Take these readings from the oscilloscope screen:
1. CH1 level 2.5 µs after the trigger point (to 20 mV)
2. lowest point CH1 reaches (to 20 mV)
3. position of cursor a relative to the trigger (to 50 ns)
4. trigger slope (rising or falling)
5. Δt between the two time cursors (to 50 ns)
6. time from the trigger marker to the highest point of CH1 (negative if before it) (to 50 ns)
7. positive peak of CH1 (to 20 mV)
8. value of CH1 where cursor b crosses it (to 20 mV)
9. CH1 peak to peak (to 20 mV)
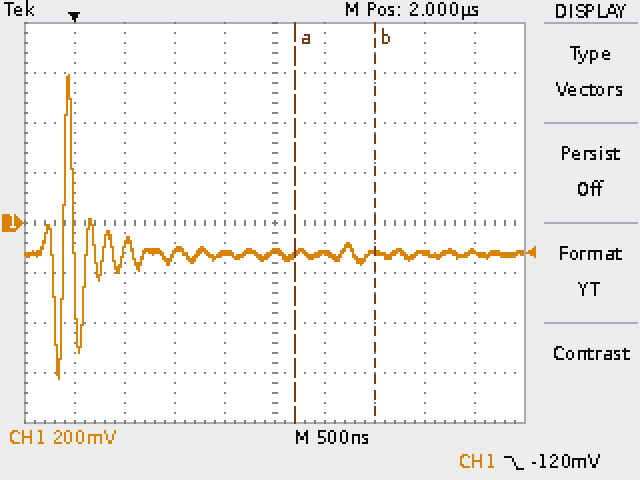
-120 mV
-620 mV
+2.20 µs
falling
800 ns
-50 ns
600 mV
-120 mV
1.22 V
